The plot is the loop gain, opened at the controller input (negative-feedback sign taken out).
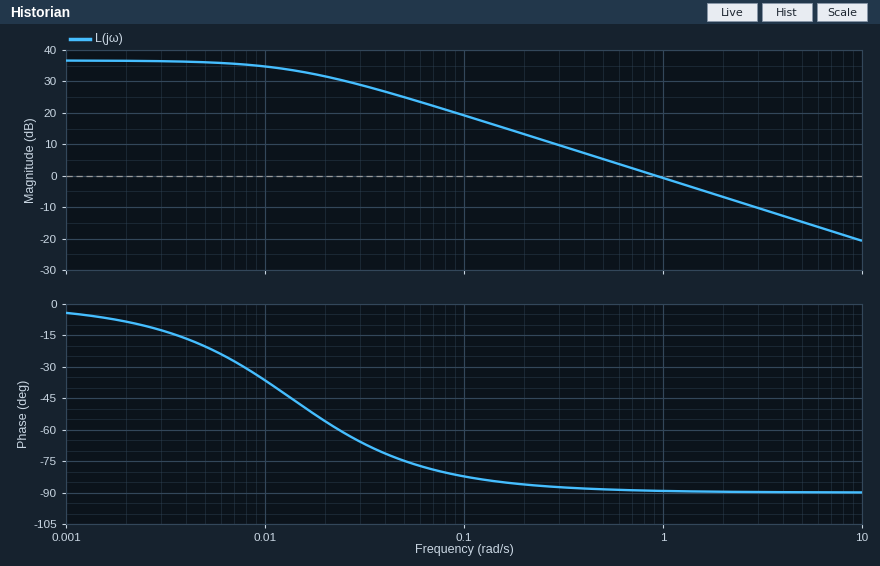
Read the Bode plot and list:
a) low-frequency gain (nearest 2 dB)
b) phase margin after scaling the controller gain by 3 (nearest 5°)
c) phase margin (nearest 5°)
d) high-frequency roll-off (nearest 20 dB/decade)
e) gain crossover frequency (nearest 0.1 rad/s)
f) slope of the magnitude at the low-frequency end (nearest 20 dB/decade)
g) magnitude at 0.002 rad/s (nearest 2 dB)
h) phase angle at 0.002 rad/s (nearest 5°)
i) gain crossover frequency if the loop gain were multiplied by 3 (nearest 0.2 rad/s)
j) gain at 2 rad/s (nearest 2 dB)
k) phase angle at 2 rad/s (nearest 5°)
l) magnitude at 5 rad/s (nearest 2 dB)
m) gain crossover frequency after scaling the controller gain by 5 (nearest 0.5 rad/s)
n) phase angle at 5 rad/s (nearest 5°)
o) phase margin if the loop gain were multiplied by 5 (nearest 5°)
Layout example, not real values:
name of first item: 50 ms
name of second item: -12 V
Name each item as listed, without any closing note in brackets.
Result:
low-frequency gain: 36 dB
phase margin after scaling the controller gain by 3: 90°
phase margin: 90°
high-frequency roll-off: -20 dB/decade
gain crossover frequency: 0.9 rad/s
slope of the magnitude at the low-frequency end: 0 dB/decade
magnitude at 0.002 rad/s: 36 dB
phase angle at 0.002 rad/s: -10°
gain crossover frequency if the loop gain were multiplied by 3: 2.8 rad/s
gain at 2 rad/s: -6 dB
phase angle at 2 rad/s: -90°
magnitude at 5 rad/s: -14 dB
gain crossover frequency after scaling the controller gain by 5: 4.5 rad/s
phase angle at 5 rad/s: -90°
phase margin if the loop gain were multiplied by 5: 90°
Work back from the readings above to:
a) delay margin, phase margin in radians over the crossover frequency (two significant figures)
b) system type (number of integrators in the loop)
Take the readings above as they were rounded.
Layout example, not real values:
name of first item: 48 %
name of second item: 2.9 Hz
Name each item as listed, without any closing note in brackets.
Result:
delay margin, phase margin in radians over the crossover frequency: 1.7 s
system type: 0
